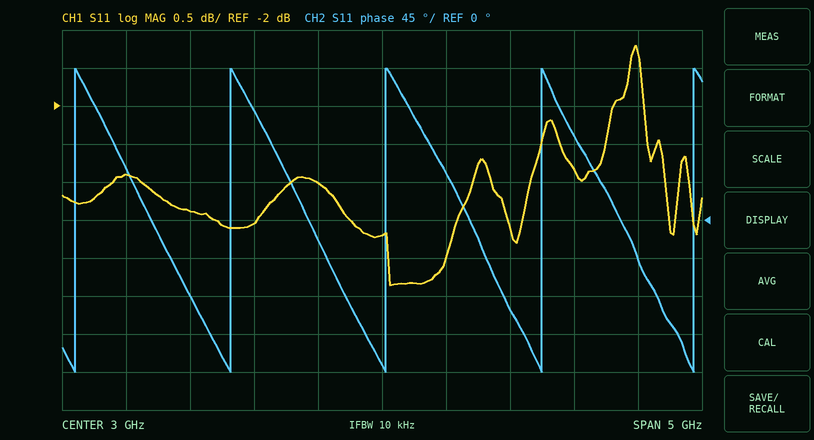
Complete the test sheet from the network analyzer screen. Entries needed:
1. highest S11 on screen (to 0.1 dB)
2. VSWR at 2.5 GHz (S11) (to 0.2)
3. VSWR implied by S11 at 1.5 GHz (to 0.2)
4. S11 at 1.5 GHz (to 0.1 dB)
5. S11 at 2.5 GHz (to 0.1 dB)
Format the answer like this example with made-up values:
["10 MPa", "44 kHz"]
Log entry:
["-1.2 dB", "5.8", "5.2", "-3.4 dB", "-3.0 dB"]
